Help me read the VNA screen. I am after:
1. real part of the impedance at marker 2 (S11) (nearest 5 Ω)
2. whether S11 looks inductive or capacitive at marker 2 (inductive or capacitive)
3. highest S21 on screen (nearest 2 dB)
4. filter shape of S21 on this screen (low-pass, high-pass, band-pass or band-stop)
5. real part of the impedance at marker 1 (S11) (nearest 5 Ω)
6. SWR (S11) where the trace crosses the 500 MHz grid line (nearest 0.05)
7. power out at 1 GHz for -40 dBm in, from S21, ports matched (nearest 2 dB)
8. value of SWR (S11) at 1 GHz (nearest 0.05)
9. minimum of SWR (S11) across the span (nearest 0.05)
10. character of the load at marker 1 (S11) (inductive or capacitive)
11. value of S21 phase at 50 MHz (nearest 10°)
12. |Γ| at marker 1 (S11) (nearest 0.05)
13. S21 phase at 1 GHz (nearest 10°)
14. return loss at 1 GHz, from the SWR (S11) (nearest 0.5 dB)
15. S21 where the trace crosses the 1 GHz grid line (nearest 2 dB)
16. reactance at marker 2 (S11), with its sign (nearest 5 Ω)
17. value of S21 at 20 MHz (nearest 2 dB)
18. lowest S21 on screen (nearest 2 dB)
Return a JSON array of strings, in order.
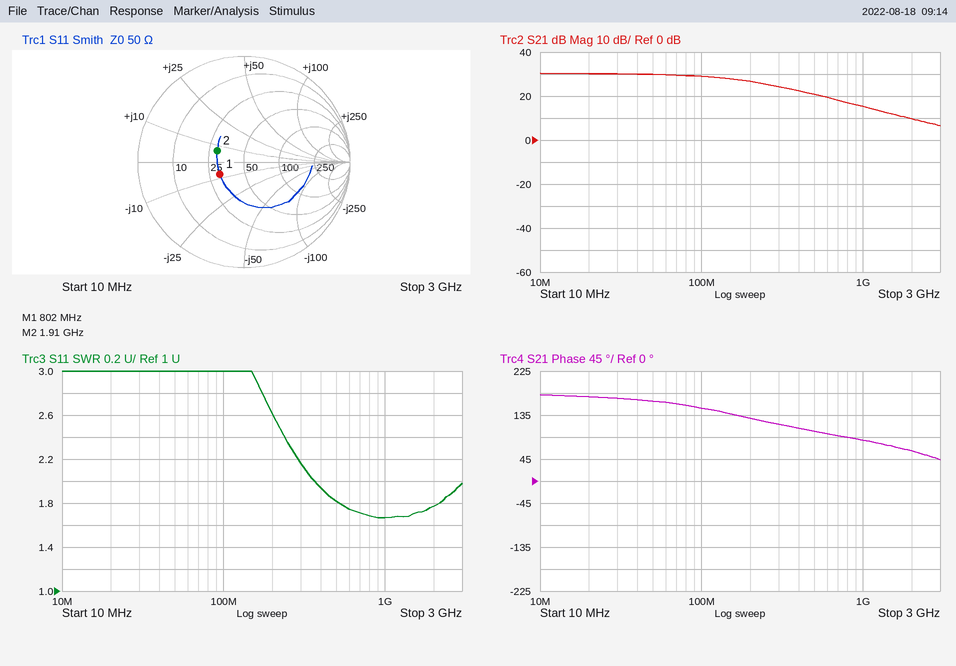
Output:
["30 Ω", "inductive", "30 dB", "low-pass", "30 Ω", "1.80", "-24 dBm", "1.65", "1.65", "capacitive", "160°", "0.25", "80°", "12.0 dB", "16 dB", "+5 Ω", "30 dB", "6 dB"]
